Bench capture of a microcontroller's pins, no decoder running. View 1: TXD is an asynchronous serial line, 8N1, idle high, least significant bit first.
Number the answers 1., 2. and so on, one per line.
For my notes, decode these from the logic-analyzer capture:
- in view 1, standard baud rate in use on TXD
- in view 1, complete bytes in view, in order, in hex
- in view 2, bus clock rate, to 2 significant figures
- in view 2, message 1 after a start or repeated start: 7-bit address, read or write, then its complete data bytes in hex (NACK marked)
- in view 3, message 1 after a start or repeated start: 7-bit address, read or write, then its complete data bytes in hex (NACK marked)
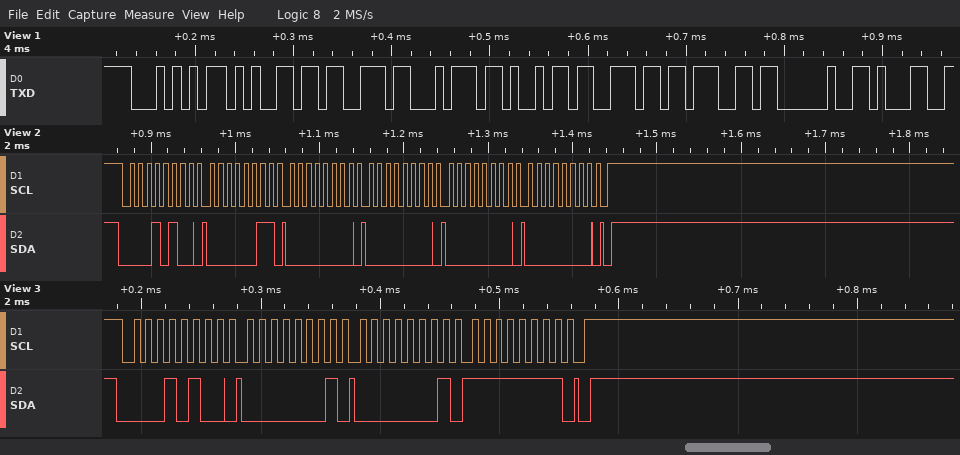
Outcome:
1. 115200 baud
2. 54 65 73 74 69 6E 67 20 31
3. 100 kHz
4. 0x0A write: 03 00 00 00 00
5. 0x0A write: 01 01 FF
